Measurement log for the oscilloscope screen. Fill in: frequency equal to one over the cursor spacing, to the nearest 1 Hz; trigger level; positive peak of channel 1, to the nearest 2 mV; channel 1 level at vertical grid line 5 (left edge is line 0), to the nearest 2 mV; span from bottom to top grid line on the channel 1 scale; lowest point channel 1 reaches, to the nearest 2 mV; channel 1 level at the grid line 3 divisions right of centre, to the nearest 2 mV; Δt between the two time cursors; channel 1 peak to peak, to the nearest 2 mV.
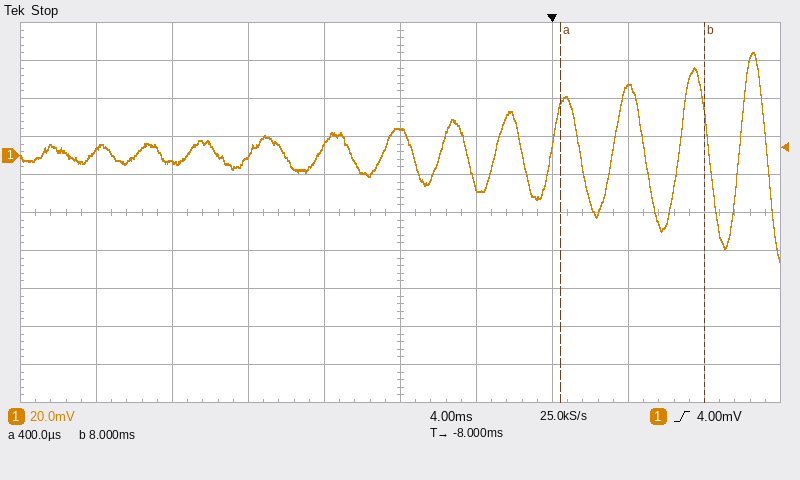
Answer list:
132 Hz
4.00 mV
54 mV
14 mV
200 mV
-56 mV
36 mV
7.6 ms
110 mV
